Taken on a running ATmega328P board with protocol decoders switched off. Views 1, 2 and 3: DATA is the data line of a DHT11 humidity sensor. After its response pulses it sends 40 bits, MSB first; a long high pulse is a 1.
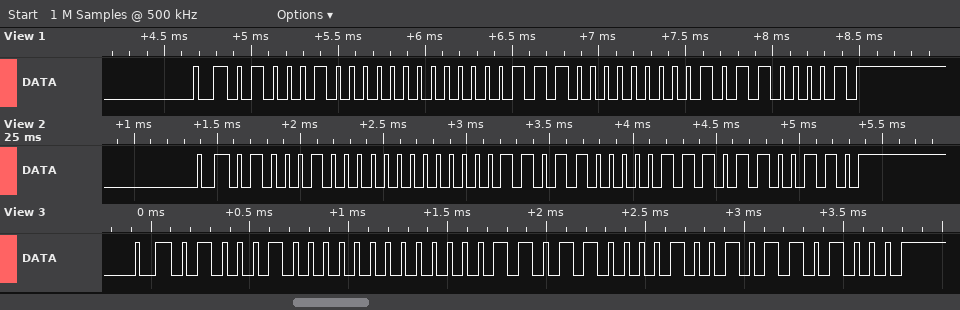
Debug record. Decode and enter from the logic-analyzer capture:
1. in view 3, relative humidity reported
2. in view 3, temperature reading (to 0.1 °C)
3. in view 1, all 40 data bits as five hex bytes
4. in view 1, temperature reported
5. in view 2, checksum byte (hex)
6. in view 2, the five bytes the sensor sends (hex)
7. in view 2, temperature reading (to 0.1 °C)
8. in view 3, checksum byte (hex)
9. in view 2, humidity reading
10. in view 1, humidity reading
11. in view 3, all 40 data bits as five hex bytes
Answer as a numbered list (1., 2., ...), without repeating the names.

1. 68 %
2. 27.9 °C
3. 44 00 1C 01 61
4. 28.1 °C
5. 0x66
6. 44 00 1B 07 66
7. 27.7 °C
8. 0x68
9. 68 %
10. 68 %
11. 44 00 1B 09 68
